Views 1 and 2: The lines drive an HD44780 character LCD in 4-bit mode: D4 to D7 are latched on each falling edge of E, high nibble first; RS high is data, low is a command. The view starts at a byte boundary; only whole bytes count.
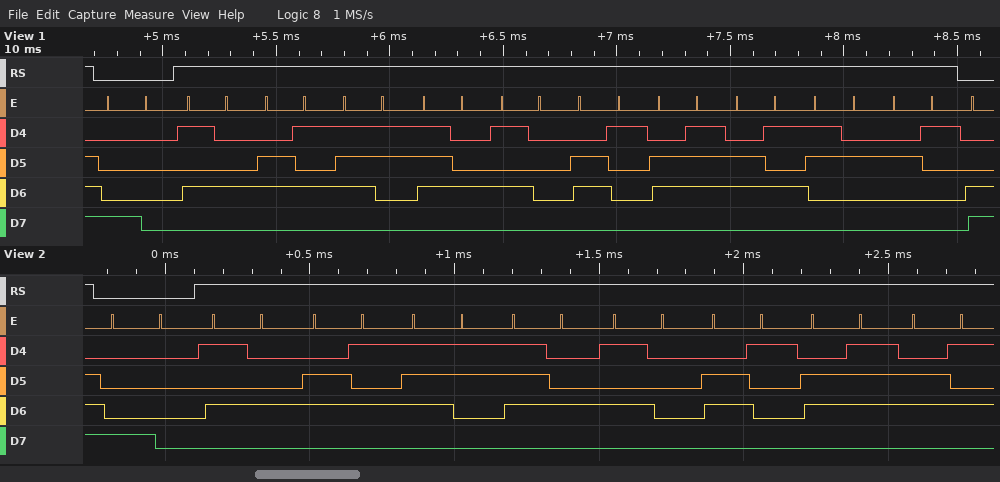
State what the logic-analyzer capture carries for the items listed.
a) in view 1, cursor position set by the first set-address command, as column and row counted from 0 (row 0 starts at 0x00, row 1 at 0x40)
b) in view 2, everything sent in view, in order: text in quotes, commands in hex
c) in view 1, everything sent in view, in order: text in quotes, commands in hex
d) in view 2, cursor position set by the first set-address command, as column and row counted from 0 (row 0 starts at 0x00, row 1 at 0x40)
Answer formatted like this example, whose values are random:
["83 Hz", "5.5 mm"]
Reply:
["column 0, row 0", "0x80 \"TestPage\"", "0x80 \"TestPage2!\"", "column 0, row 0"]
